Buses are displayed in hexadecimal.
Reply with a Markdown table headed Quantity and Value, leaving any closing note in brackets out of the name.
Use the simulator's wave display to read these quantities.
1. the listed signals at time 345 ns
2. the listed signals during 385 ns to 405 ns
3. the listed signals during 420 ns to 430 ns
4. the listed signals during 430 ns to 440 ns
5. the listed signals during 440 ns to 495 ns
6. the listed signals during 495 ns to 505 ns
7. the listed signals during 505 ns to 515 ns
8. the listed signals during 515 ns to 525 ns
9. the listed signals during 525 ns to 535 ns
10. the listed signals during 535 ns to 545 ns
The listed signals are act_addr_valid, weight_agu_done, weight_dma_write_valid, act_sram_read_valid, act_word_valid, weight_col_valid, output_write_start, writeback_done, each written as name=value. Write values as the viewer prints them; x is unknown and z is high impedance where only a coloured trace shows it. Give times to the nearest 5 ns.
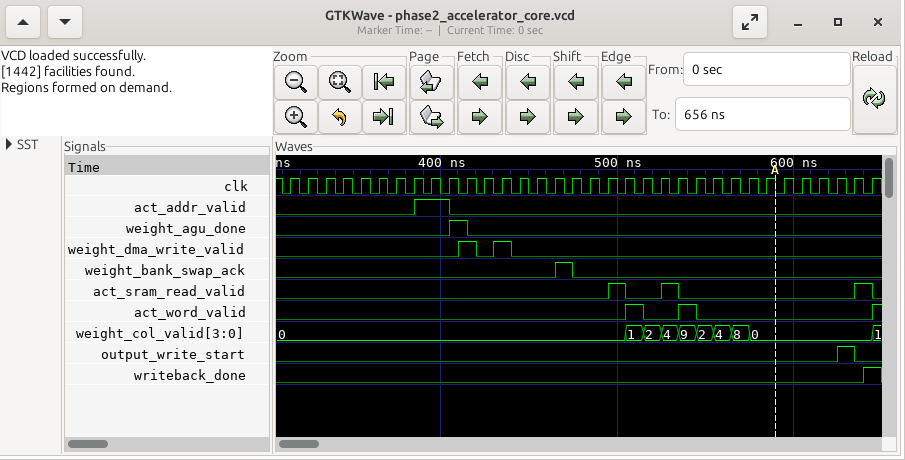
| Quantity | Value |
|---|---|
| the listed signals at time 345 ns | act_addr_valid=0, weight_agu_done=0, weight_dma_write_valid=0, act_sram_read_valid=0, act_word_valid=0, weight_col_valid=0, output_write_start=0, writeback_done=0 |
| the listed signals during 385 ns to 405 ns | act_addr_valid=1, weight_agu_done=0, weight_dma_write_valid=0, act_sram_read_valid=0, act_word_valid=0, weight_col_valid=0, output_write_start=0, writeback_done=0 |
| the listed signals during 420 ns to 430 ns | act_addr_valid=0, weight_agu_done=0, weight_dma_write_valid=0, act_sram_read_valid=0, act_word_valid=0, weight_col_valid=0, output_write_start=0, writeback_done=0 |
| the listed signals during 430 ns to 440 ns | act_addr_valid=0, weight_agu_done=0, weight_dma_write_valid=1, act_sram_read_valid=0, act_word_valid=0, weight_col_valid=0, output_write_start=0, writeback_done=0 |
| the listed signals during 440 ns to 495 ns | act_addr_valid=0, weight_agu_done=0, weight_dma_write_valid=0, act_sram_read_valid=0, act_word_valid=0, weight_col_valid=0, output_write_start=0, writeback_done=0 |
| the listed signals during 495 ns to 505 ns | act_addr_valid=0, weight_agu_done=0, weight_dma_write_valid=0, act_sram_read_valid=1, act_word_valid=0, weight_col_valid=0, output_write_start=0, writeback_done=0 |
| the listed signals during 505 ns to 515 ns | act_addr_valid=0, weight_agu_done=0, weight_dma_write_valid=0, act_sram_read_valid=0, act_word_valid=1, weight_col_valid=1, output_write_start=0, writeback_done=0 |
| the listed signals during 515 ns to 525 ns | act_addr_valid=0, weight_agu_done=0, weight_dma_write_valid=0, act_sram_read_valid=0, act_word_valid=0, weight_col_valid=2, output_write_start=0, writeback_done=0 |
| the listed signals during 525 ns to 535 ns | act_addr_valid=0, weight_agu_done=0, weight_dma_write_valid=0, act_sram_read_valid=1, act_word_valid=0, weight_col_valid=4, output_write_start=0, writeback_done=0 |
| the listed signals during 535 ns to 545 ns | act_addr_valid=0, weight_agu_done=0, weight_dma_write_valid=0, act_sram_read_valid=0, act_word_valid=1, weight_col_valid=9, output_write_start=0, writeback_done=0 |
